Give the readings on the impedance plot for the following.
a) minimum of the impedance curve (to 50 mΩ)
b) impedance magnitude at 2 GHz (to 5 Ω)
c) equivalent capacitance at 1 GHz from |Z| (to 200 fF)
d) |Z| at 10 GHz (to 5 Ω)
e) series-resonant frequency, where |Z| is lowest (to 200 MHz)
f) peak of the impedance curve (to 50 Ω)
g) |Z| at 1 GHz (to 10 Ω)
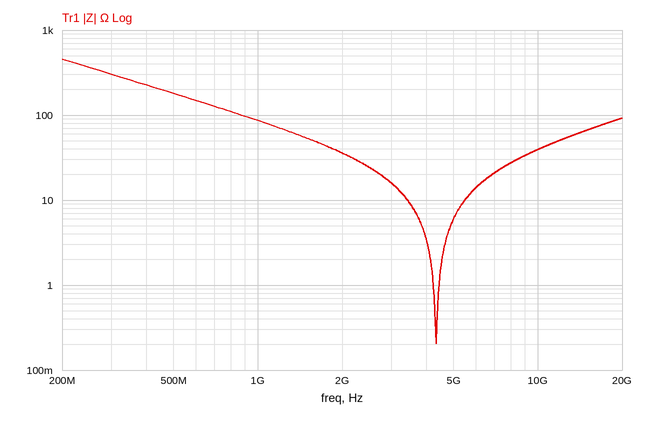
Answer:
200 mΩ
35 Ω
1.8 pF
40 Ω
4.4 GHz
450 Ω
90 Ω
